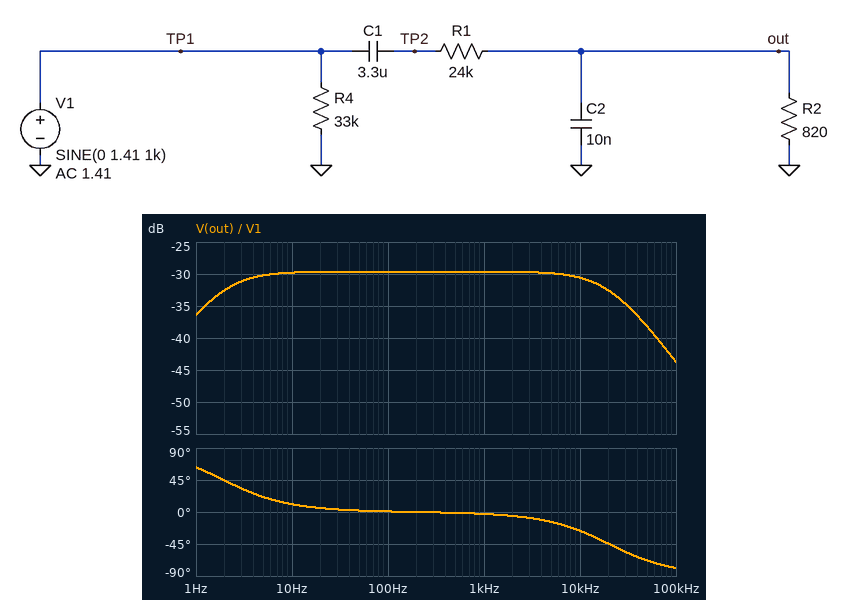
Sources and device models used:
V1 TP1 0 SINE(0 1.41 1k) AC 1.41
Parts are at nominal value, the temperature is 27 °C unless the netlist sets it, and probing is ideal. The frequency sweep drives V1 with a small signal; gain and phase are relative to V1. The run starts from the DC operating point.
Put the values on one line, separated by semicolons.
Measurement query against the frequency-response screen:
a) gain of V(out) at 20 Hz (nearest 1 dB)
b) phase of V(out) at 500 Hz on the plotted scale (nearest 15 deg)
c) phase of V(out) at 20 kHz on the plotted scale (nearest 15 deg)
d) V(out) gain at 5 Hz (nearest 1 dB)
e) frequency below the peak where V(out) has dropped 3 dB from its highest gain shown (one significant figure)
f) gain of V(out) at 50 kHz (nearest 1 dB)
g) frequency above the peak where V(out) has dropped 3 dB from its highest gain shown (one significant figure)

-30 dB; 0 deg; -45 deg; -30 dB; 2 Hz; -38 dB; 20 kHz
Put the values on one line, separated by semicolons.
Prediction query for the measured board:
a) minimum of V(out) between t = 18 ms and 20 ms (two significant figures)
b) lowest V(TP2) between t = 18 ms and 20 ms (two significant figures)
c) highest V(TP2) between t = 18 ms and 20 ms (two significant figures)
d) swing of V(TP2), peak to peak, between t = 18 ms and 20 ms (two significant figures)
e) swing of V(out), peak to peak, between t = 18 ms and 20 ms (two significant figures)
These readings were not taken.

-47 mV; -1.4 V; 1.4 V; 2.8 V; 93 mV
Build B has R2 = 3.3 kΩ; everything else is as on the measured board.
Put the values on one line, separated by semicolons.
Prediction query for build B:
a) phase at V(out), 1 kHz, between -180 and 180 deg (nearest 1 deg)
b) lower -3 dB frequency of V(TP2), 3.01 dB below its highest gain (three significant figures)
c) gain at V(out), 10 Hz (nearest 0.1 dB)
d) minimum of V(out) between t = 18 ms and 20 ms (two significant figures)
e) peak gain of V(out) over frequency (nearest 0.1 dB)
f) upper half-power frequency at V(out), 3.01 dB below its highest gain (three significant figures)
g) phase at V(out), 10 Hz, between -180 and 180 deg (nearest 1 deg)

-10 deg; 1.77 Hz; -18.5 dB; -170 mV; -18.4 dB; 5.49 kHz; 10 deg
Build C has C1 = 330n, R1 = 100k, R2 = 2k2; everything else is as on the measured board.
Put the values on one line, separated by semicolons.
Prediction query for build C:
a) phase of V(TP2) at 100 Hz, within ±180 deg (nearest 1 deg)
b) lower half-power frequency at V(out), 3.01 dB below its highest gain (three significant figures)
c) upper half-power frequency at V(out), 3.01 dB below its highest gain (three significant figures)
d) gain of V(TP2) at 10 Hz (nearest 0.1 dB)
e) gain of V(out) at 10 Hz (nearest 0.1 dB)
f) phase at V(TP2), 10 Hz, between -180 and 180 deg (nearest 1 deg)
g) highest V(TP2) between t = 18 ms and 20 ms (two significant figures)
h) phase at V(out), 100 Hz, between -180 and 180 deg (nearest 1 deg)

3 deg; 4.71 Hz; 7.40 kHz; -0.9 dB; -34.2 dB; 25 deg; 1.4 V; 2 deg
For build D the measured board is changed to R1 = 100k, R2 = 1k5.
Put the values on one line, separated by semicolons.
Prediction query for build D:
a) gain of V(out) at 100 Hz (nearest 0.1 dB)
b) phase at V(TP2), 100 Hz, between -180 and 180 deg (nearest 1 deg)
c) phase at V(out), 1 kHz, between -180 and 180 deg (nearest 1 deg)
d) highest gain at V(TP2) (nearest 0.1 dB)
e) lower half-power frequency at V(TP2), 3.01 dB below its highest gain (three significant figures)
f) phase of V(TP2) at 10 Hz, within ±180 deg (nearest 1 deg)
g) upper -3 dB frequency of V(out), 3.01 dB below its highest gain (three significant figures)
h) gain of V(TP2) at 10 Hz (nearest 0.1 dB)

-36.6 dB; 0 deg; -5 deg; 0 dB; 475 mHz; 3 deg; 10.8 kHz; 0 dB
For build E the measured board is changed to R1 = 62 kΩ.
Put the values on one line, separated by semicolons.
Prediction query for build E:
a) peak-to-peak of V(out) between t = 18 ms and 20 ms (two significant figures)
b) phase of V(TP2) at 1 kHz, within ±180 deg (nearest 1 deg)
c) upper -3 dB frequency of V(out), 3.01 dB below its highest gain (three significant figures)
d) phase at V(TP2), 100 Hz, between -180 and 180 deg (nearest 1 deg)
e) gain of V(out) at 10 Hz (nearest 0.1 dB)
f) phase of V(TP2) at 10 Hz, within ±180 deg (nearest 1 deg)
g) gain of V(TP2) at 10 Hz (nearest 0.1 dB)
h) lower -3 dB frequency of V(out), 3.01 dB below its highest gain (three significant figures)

37 mV; 0 deg; 19.7 kHz; 0 deg; -37.7 dB; 4 deg; 0 dB; 768 mHz
